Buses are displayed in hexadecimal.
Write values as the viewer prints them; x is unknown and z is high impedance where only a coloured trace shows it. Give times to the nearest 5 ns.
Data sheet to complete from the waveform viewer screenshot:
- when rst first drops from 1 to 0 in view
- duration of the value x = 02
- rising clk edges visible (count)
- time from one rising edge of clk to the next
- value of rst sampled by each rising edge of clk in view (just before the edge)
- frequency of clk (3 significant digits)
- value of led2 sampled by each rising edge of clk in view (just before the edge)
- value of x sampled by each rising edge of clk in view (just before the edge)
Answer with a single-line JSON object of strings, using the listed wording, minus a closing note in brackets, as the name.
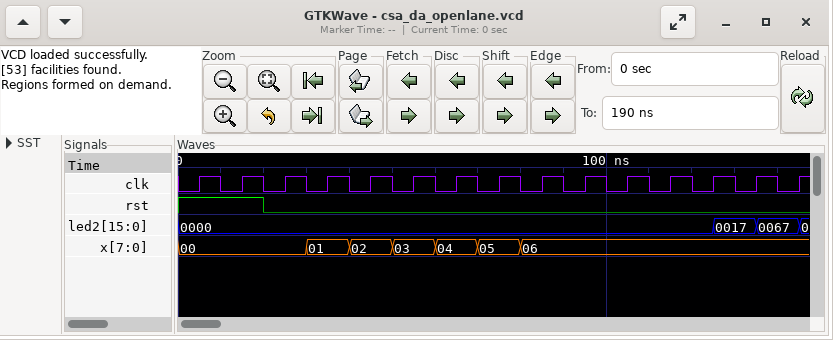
{"when rst first drops from 1 to 0 in view": "20 ns", "duration of the value x = 02": "10 ns", "rising clk edges visible": "15", "time from one rising edge of clk to the next": "10 ns", "value of rst sampled by each rising edge of clk in view": "1 1 0 0 0 0 0 0 0 0 0 0 0 0 0", "frequency of clk": "100 MHz", "value of led2 sampled by each rising edge of clk in view": "0000, 0000, 0000, 0000, 0000, 0000, 0000, 0000, 0000, 0000, 0000, 0000, 0000, 0017, 0067", "value of x sampled by each rising edge of clk in view": "00, 00, 00, 01, 02, 03, 04, 05, 06, 06, 06, 06, 06, 06, 06"}
